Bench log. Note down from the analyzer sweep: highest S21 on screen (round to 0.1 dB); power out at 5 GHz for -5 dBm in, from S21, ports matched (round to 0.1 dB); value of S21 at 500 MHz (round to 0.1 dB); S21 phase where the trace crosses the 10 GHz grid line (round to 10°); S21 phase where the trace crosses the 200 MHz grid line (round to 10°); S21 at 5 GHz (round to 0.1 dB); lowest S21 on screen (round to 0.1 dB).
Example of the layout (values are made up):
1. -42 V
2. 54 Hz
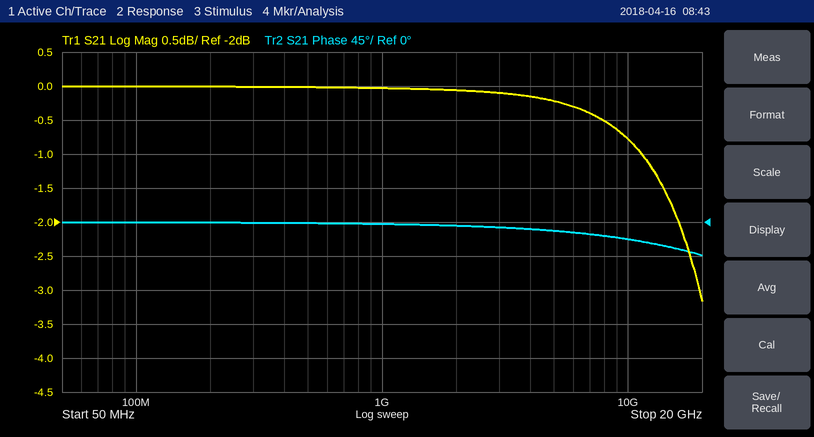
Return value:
1. 0.0 dB
2. -5.2 dBm
3. 0.0 dB
4. -20°
5. 0°
6. -0.2 dB
7. -3.2 dB
